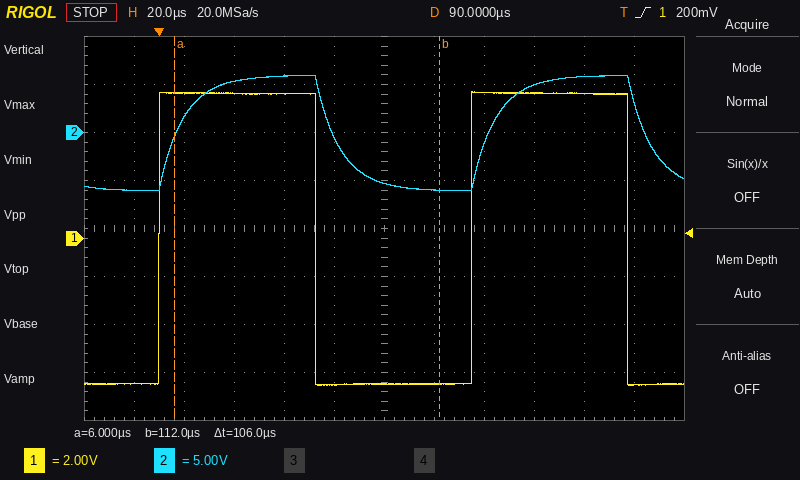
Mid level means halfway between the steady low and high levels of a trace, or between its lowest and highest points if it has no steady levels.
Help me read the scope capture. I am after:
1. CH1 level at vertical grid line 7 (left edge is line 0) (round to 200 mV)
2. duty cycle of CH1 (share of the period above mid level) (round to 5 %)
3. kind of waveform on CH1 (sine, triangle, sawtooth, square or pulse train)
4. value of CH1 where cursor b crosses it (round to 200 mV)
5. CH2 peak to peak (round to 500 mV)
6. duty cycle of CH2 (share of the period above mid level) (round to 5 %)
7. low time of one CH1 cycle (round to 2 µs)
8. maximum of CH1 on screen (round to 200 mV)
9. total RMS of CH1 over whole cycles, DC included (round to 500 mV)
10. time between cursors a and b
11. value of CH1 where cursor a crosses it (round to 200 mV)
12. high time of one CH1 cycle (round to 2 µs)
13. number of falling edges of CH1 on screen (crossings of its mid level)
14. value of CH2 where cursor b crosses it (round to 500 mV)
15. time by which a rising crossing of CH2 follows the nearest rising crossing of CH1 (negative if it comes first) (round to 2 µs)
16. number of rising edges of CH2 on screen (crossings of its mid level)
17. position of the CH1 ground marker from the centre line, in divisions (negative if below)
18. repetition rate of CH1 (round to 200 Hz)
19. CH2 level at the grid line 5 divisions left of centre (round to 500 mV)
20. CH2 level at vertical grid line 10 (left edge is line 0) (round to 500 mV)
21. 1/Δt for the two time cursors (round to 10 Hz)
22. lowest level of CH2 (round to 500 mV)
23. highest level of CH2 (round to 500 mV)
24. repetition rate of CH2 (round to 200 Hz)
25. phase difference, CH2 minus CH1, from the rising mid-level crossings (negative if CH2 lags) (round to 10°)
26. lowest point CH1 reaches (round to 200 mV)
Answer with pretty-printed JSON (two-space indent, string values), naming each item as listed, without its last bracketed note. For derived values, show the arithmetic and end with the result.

{
  "CH1 level at vertical grid line 7 (left edge is line 0)": "-6.0 V",
  "duty cycle of CH1 (share of the period above mid level)": "50 %",
  "kind of waveform on CH1": "square",
  "value of CH1 where cursor b crosses it": "-6.0 V",
  "CH2 peak to peak": "6.0 V − (-6.0 V) = 12.0 V",
  "duty cycle of CH2 (share of the period above mid level)": "50 %",
  "low time of one CH1 cycle": "62 µs",
  "maximum of CH1 on screen": "6.2 V",
  "total RMS of CH1 over whole cycles, DC included": "√(0.5 × (6.2 V)² + 0.5 × (-6.2 V)²) ≈ 6.20 V, so 6.0 V to the nearest 500 mV",
  "time between cursors a and b": "106 µs",
  "value of CH1 where cursor a crosses it": "6.0 V",
  "high time of one CH1 cycle": "62 µs",
  "number of falling edges of CH1 on screen": "2",
  "value of CH2 where cursor b crosses it": "-6.0 V",
  "time by which a rising crossing of CH2 follows the nearest rising crossing of CH1 (negative if it comes first)": "+6 µs",
  "number of rising edges of CH2 on screen": "2",
  "position of the CH1 ground marker from the centre line, in divisions": "-0.2 div",
  "repetition rate of CH1": "8.0 kHz",
  "CH2 level at the grid line 5 divisions left of centre": "-6.0 V",
  "CH2 level at vertical grid line 10 (left edge is line 0)": "6.0 V",
  "1/Δt for the two time cursors": "1 / 106 µs ≈ 9.43 kHz",
  "lowest level of CH2": "-6.0 V",
  "highest level of CH2": "6.0 V",
  "repetition rate of CH2": "8.0 kHz",
  "phase difference, CH2 minus CH1, from the rising mid-level crossings (negative if CH2 lags)": "-20°",
  "lowest point CH1 reaches": "-6.2 V"
}
